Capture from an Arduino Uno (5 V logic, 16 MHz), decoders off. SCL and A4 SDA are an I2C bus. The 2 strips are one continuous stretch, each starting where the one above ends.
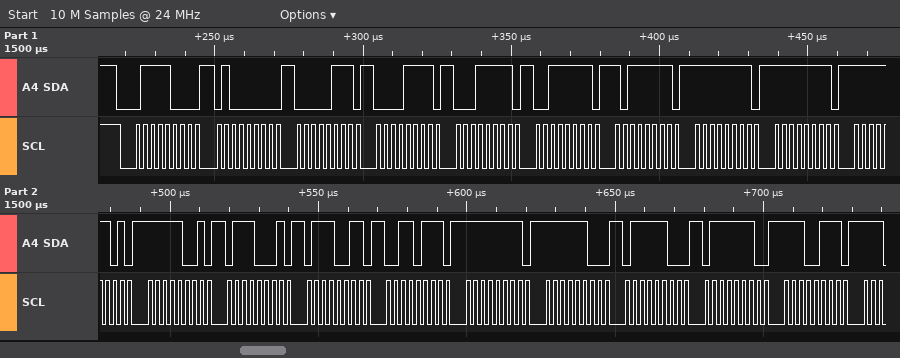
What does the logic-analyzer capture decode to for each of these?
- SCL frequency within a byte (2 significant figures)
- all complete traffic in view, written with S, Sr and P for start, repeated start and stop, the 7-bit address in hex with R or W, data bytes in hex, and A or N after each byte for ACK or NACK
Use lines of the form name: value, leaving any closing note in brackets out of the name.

SCL frequency within a byte: 400 kHz
all complete traffic in view, written with S, Sr and P for start, repeated start and stop, the 7-bit address in hex with R or W, data bytes in hex, and A or N after each byte for ACK or NACK: S 3CW A 40 A 07 A 0F A 1F A 3F A BF A FF A FF A FD A F9 A 71 A 73 A 37 A FF A FC A 7C A 7E A E7 A
